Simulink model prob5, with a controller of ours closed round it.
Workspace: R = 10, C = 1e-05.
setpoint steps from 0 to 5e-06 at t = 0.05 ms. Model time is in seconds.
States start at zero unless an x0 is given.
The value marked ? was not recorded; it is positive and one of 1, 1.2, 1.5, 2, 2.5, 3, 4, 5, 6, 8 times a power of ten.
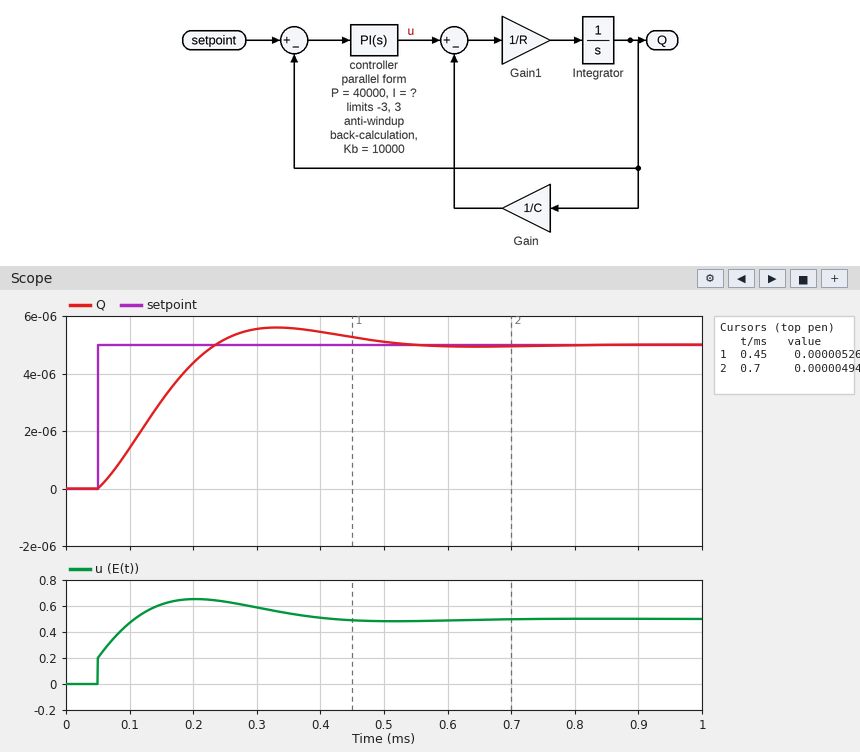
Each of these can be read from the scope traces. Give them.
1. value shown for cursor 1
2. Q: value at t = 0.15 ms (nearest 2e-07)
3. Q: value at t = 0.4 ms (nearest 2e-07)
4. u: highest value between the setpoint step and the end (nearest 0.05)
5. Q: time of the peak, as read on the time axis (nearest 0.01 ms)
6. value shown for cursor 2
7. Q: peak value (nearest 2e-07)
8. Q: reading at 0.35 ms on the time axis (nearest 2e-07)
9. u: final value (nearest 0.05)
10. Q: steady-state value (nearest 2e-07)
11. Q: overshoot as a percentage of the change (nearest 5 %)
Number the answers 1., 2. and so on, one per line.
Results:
1. 0.00000526
2. 0.0000030
3. 0.0000054
4. 0.65
5. 0.33 ms
6. 0.00000494
7. 0.0000056
8. 0.0000056
9. 0.50
10. 0.0000050
11. 10 %
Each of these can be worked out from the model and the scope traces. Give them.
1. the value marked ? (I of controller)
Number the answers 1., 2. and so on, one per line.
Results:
1. 1.5e+09
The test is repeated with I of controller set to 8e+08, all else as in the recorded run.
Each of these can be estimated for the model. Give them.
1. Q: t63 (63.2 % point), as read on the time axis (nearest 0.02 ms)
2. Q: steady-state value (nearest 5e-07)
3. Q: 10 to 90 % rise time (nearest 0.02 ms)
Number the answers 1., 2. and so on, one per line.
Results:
1. 0.20 ms
2. 0.0000050
3. 0.24 ms
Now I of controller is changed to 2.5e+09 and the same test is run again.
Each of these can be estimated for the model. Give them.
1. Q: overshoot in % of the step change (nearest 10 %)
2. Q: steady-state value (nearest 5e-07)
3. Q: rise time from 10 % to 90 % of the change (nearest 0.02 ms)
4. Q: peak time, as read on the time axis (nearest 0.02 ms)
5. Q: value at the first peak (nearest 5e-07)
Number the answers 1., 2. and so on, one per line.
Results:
1. 20 %
2. 0.0000050
3. 0.10 ms
4. 0.26 ms
5. 0.0000060
